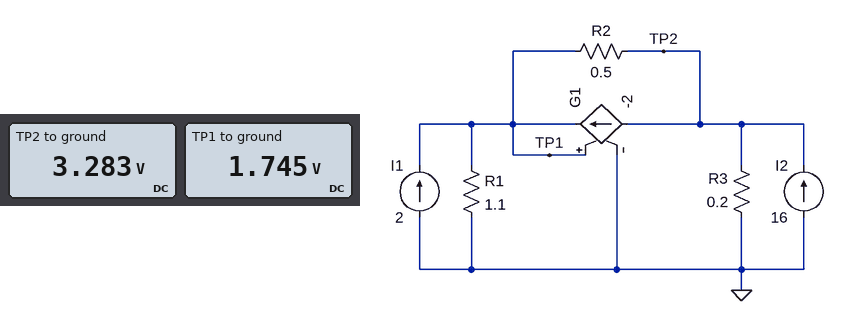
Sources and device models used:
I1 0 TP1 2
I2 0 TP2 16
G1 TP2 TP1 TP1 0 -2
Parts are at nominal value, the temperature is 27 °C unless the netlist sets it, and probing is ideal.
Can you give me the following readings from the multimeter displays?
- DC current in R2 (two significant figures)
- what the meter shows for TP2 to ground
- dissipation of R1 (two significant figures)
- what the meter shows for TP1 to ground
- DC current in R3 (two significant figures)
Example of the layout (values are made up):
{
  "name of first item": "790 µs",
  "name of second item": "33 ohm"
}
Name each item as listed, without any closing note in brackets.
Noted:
{
  "DC current in R2": "3.1 A",
  "what the meter shows for TP2 to ground": "3.283 V",
  "dissipation of R1": "2.8 W",
  "what the meter shows for TP1 to ground": "1.745 V",
  "DC current in R3": "16 A"
}
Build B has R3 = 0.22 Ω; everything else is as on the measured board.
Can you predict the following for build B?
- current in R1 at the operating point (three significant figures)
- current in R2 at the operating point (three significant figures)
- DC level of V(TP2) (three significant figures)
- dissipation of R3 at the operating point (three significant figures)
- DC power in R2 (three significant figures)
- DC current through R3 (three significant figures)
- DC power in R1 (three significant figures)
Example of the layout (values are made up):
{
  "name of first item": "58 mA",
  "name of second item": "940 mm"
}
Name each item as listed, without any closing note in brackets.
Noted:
{
  "current in R1 at the operating point": "1.70 A",
  "current in R2 at the operating point": "3.44 A",
  "DC level of V(TP2)": "3.59 V",
  "dissipation of R3 at the operating point": "58.5 W",
  "DC power in R2": "5.90 W",
  "DC current through R3": "16.3 A",
  "DC power in R1": "3.17 W"
}
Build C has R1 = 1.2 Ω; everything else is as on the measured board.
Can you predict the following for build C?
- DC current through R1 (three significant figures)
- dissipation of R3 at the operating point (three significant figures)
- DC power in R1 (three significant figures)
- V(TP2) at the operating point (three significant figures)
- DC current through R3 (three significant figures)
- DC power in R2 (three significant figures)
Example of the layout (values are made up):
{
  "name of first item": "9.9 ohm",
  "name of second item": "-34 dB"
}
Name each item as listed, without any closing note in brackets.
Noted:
{
  "DC current through R1": "1.48 A",
  "dissipation of R3 at the operating point": "54.6 W",
  "DC power in R1": "2.64 W",
  "V(TP2) at the operating point": "3.30 V",
  "DC current through R3": "16.5 A",
  "DC power in R2": "4.64 W"
}
